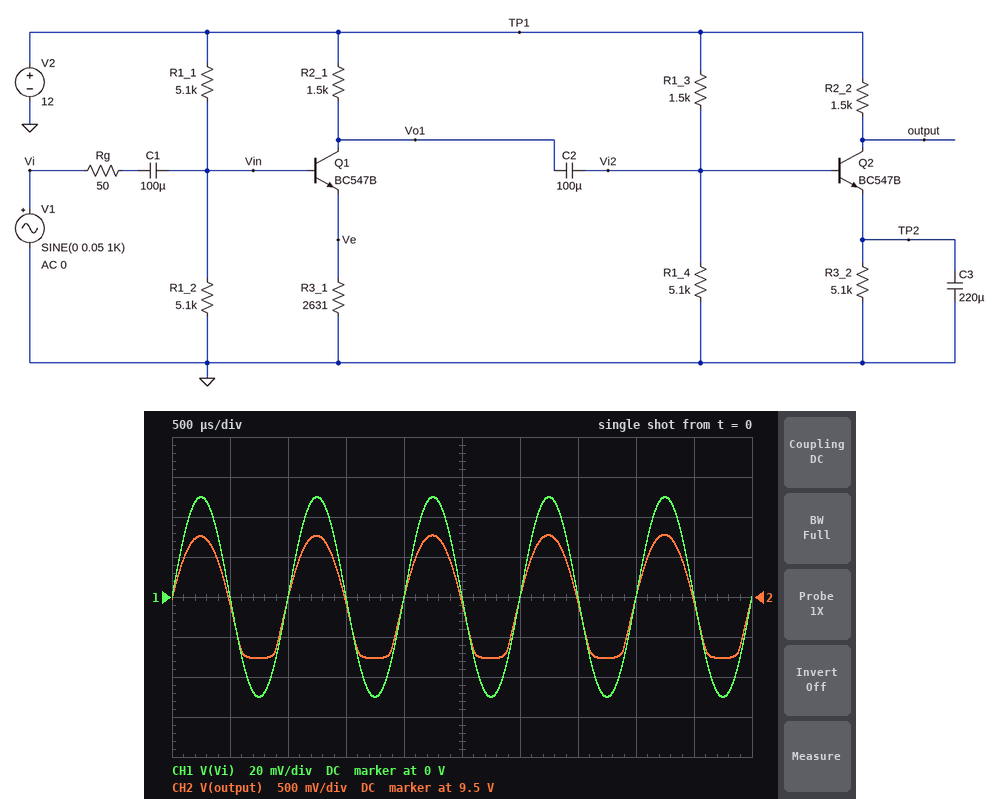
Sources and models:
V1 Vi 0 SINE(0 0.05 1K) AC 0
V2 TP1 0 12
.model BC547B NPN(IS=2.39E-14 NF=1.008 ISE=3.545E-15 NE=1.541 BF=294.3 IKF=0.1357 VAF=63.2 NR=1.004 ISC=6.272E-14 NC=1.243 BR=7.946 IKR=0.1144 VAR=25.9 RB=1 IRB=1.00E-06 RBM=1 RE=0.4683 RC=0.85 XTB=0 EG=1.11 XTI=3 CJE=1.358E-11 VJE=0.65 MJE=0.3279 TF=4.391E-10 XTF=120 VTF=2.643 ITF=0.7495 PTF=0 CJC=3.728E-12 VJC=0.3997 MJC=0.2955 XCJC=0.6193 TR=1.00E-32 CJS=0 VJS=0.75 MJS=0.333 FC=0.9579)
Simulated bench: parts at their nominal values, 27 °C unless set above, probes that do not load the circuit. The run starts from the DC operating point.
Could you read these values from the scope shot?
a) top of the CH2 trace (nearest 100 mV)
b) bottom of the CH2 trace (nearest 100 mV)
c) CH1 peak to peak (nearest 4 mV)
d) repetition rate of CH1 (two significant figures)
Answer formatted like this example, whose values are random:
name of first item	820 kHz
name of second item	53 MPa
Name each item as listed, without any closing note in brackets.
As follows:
top of the CH2 trace	10.3 V
bottom of the CH2 trace	8.7 V
CH1 peak to peak	100 mV
repetition rate of CH1	1.0 kHz
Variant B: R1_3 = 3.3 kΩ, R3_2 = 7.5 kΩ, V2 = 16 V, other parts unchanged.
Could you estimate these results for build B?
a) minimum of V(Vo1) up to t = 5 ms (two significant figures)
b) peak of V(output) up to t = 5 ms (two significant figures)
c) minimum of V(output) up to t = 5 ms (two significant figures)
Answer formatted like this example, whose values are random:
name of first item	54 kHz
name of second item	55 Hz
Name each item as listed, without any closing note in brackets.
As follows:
minimum of V(Vo1) up to t = 5 ms	12 V
peak of V(output) up to t = 5 ms	15 V
minimum of V(output) up to t = 5 ms	13 V
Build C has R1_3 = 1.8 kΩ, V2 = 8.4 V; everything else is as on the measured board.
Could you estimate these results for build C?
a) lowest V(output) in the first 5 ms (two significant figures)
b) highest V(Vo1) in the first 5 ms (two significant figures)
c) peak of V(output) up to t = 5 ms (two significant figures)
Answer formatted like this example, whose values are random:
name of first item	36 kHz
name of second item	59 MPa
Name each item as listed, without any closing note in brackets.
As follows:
lowest V(output) in the first 5 ms	5.9 V
highest V(Vo1) in the first 5 ms	6.4 V
peak of V(output) up to t = 5 ms	7.4 V
